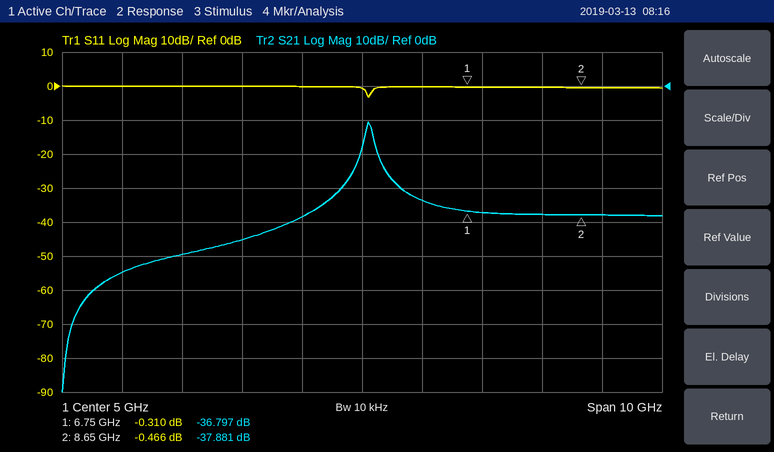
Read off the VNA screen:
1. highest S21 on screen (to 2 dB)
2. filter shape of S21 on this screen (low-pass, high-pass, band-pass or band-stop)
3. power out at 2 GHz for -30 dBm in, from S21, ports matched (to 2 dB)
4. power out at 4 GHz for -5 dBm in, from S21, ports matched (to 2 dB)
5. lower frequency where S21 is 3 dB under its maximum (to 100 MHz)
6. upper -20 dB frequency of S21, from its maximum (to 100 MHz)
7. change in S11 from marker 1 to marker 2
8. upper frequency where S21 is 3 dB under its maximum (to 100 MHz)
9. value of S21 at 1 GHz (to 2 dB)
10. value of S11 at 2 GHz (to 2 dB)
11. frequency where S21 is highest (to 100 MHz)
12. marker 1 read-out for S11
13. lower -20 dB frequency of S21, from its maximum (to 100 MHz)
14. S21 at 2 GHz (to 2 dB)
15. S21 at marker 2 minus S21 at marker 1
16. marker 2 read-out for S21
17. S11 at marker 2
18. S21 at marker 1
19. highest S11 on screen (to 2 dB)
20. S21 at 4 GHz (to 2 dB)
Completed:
-10 dB
band-pass
-80 dBm
-44 dBm
5.1 GHz
5.7 GHz
-0.156 dB
5.2 GHz
-54 dB
0 dB
5.1 GHz
-0.310 dB
4.6 GHz
-50 dB
-1.084 dB
-37.881 dB
-0.466 dB
-36.797 dB
0 dB
-38 dB
